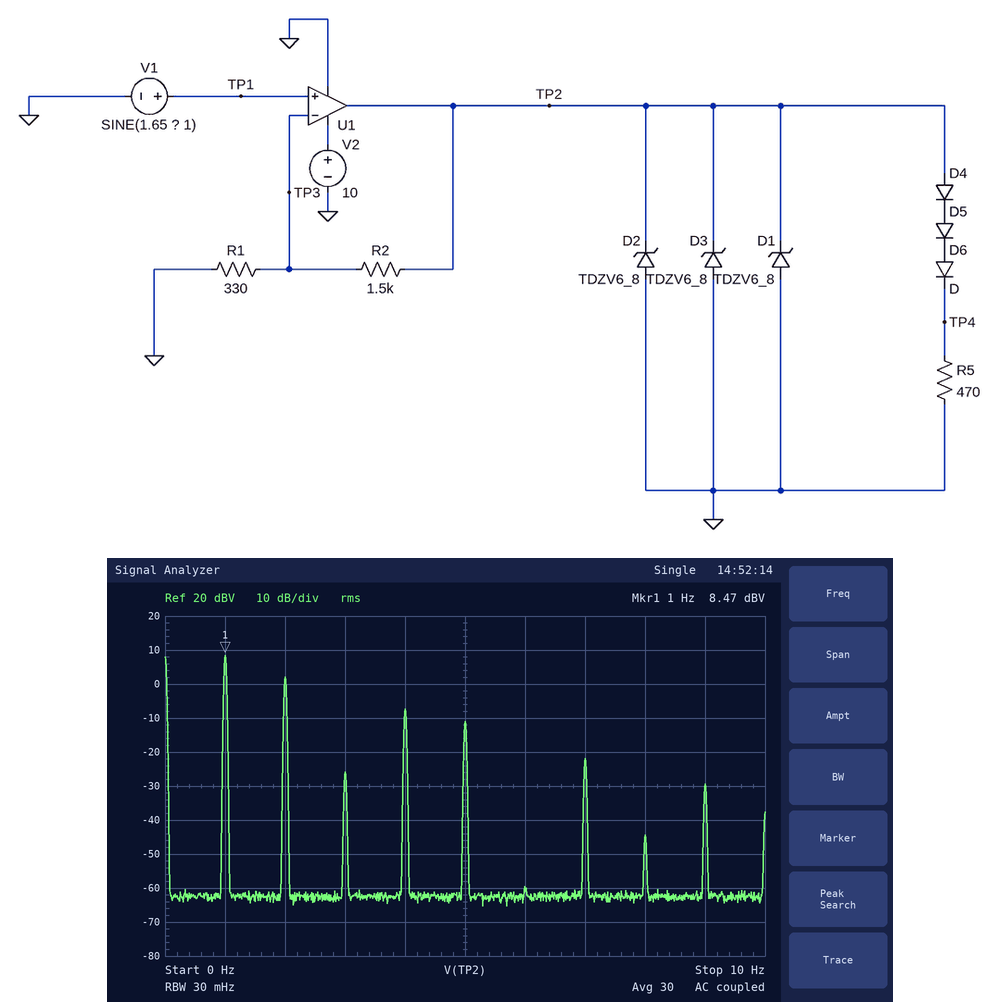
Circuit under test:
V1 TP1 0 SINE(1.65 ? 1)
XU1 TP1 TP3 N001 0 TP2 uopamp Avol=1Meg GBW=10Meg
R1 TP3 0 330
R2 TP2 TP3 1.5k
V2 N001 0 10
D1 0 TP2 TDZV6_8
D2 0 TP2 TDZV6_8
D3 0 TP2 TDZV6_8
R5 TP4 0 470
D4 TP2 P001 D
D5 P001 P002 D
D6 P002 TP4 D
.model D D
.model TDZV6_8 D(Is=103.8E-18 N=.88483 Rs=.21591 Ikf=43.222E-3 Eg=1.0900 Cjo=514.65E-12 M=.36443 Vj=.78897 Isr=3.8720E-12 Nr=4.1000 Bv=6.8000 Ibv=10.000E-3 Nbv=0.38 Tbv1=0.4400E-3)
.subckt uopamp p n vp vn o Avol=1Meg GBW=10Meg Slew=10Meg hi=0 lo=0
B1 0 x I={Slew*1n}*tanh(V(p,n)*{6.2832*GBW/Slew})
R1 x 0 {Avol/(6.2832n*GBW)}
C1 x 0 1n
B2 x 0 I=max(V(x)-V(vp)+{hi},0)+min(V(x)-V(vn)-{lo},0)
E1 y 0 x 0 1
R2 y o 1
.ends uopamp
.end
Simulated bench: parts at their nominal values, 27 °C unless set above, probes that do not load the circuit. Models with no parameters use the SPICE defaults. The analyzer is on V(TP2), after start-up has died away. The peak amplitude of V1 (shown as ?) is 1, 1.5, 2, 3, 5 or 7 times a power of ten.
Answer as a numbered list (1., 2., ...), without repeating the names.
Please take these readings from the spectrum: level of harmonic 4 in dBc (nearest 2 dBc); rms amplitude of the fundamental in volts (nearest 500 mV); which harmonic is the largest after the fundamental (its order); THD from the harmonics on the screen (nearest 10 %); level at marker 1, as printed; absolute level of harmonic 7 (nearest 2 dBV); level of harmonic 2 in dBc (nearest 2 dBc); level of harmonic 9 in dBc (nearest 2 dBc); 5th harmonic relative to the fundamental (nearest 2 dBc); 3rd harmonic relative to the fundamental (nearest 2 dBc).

1. -16 dBc
2. 2.5 V
3. 2
4. 50 %
5. 8.47 dBV
6. -22 dBV
7. -6 dBc
8. -38 dBc
9. -20 dBc
10. -34 dBc
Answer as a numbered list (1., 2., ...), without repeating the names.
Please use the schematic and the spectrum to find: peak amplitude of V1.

1. 2 V
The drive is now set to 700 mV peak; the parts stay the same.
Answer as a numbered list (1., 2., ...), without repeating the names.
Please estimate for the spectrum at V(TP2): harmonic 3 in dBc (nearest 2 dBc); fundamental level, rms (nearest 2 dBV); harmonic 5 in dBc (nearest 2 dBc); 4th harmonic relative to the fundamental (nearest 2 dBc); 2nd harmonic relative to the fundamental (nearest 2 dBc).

1. -8 dBc
2. -6 dBV
3. -26 dBc
4. -20 dBc
5. -2 dBc
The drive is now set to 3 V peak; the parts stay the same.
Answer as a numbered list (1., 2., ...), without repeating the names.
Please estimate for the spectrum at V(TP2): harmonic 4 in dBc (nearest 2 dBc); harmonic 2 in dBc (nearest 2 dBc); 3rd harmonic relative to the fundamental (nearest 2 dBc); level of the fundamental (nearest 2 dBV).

1. -12 dBc
2. -10 dBc
3. -16 dBc
4. 10 dBV
